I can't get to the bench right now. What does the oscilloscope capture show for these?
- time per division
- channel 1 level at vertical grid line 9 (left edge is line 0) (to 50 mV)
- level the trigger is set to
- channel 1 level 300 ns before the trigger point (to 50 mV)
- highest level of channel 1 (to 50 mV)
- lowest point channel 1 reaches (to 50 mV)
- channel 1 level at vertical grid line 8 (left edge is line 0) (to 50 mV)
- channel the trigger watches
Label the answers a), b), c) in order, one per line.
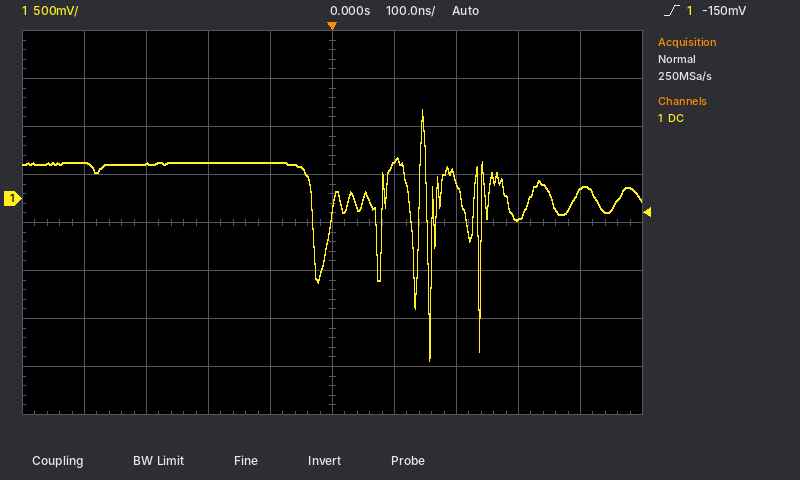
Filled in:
a) 100 ns
b) 100 mV
c) -150 mV
d) 350 mV
e) 950 mV
f) -1.70 V
g) -200 mV
h) channel 1
